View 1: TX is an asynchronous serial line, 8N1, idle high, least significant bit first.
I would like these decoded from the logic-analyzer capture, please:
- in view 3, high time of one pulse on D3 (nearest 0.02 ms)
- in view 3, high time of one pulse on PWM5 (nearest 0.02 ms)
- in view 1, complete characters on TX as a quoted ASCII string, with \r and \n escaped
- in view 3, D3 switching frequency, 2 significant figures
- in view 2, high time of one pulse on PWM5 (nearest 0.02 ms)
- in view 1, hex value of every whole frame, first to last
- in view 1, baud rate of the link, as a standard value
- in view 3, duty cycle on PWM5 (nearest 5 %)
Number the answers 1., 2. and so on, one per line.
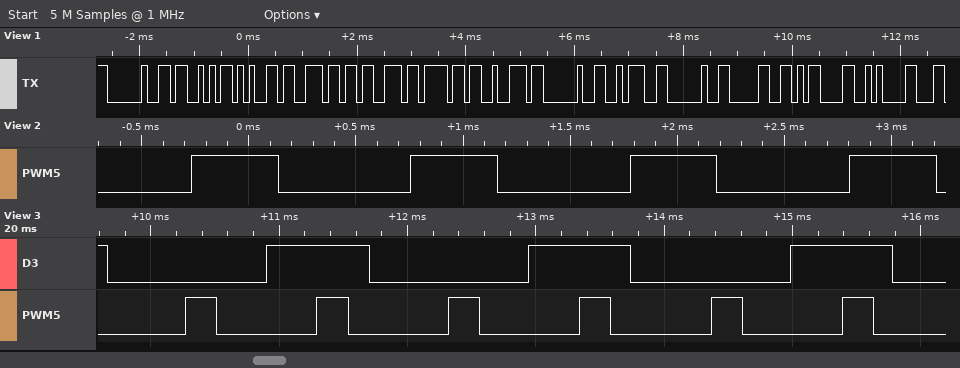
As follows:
1. 0.80 ms
2. 0.24 ms
3. " Sensor : 0\r\n"
4. 490 Hz
5. 0.40 ms
6. 20 53 65 6E 73 6F 72 20 3A 20 30 0D 0A
7. 9600 baud
8. 25 %
